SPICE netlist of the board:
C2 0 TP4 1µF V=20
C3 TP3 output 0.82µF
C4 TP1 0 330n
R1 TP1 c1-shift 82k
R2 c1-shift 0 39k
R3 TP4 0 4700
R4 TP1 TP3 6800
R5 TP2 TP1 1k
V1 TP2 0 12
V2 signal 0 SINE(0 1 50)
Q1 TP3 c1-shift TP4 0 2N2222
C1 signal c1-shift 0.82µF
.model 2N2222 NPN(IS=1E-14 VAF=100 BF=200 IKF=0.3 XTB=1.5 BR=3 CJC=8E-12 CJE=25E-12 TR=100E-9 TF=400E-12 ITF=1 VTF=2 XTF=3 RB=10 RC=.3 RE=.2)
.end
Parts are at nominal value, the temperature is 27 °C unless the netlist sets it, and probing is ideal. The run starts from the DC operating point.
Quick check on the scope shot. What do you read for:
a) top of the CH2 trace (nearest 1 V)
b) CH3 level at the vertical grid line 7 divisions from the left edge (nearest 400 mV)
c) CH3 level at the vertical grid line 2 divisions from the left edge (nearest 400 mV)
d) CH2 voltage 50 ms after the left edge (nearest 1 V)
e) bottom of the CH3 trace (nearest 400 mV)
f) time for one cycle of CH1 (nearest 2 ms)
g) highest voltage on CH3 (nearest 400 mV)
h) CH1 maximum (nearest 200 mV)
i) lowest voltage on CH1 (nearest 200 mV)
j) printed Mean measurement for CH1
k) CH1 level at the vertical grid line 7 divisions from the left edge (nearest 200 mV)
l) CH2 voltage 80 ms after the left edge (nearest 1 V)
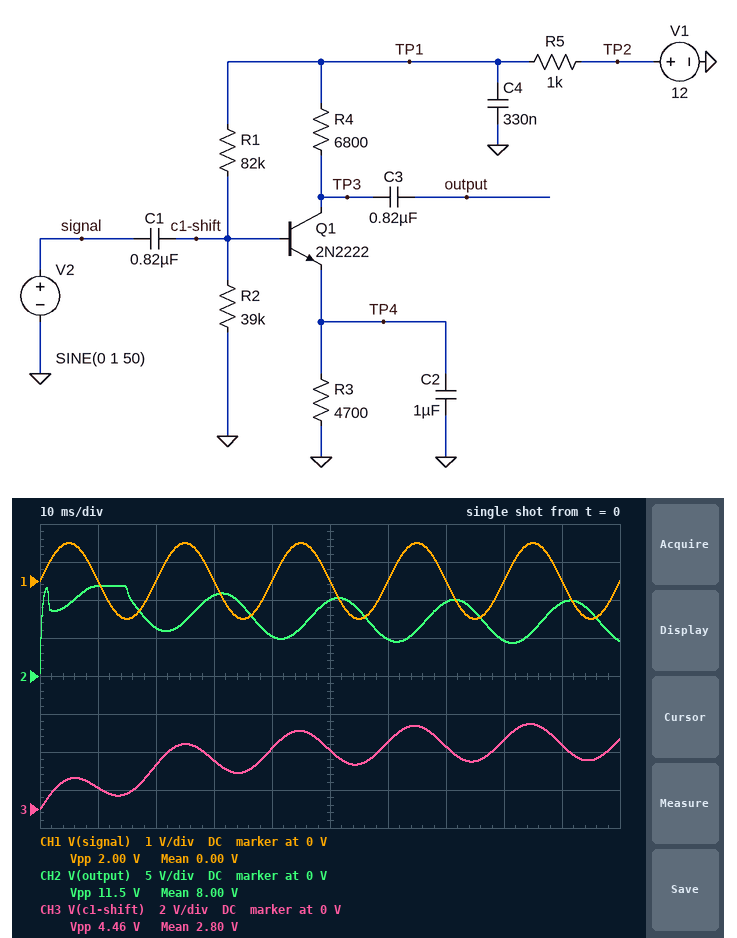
12 V
3.2 V
2.4 V
10 V
0 V
20 ms
4.4 V
1.0 V
-1.0 V
0.00 V
0 V
5 V
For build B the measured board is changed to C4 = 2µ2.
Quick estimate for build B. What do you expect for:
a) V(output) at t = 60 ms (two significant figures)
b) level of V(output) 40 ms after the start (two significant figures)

5.0 V
5.4 V
